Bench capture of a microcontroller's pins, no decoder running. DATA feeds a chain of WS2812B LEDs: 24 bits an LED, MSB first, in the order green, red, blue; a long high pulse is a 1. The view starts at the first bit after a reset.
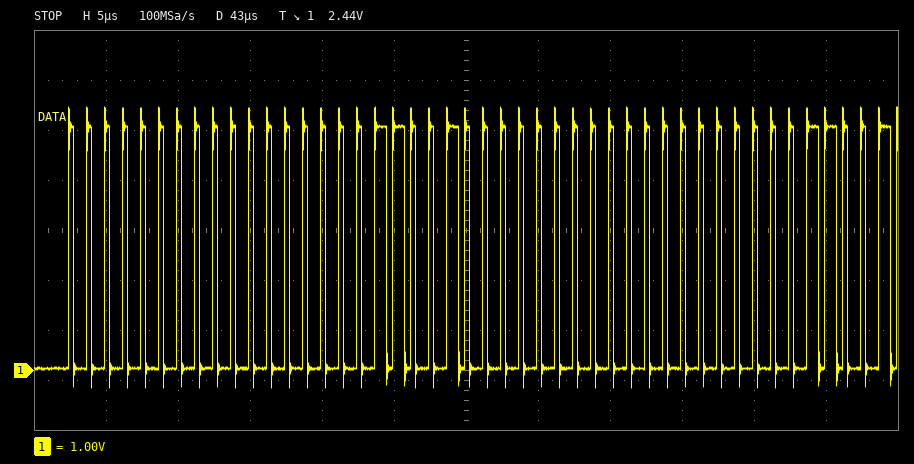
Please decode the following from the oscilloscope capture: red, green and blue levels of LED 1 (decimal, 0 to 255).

0, 0, 100
